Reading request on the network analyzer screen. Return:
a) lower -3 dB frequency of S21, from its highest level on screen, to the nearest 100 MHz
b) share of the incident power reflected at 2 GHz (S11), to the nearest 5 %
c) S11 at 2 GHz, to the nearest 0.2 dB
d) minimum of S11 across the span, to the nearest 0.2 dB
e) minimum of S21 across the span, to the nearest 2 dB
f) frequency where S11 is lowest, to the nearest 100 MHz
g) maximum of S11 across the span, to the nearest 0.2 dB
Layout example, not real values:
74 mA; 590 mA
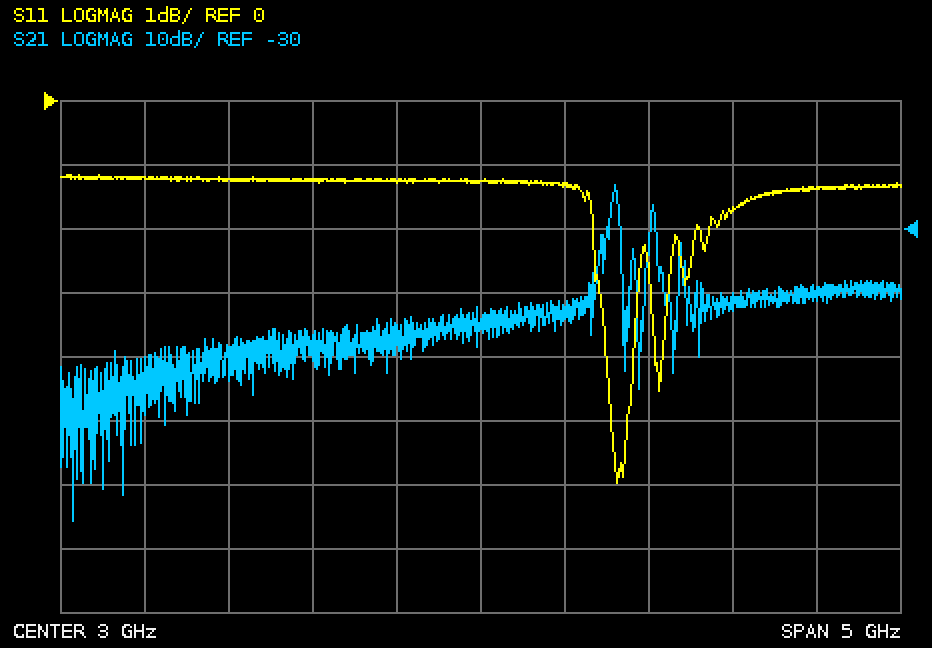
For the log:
3.8 GHz; 75 %; -1.2 dB; -6.0 dB; -76 dB; 3.8 GHz; -1.2 dB
